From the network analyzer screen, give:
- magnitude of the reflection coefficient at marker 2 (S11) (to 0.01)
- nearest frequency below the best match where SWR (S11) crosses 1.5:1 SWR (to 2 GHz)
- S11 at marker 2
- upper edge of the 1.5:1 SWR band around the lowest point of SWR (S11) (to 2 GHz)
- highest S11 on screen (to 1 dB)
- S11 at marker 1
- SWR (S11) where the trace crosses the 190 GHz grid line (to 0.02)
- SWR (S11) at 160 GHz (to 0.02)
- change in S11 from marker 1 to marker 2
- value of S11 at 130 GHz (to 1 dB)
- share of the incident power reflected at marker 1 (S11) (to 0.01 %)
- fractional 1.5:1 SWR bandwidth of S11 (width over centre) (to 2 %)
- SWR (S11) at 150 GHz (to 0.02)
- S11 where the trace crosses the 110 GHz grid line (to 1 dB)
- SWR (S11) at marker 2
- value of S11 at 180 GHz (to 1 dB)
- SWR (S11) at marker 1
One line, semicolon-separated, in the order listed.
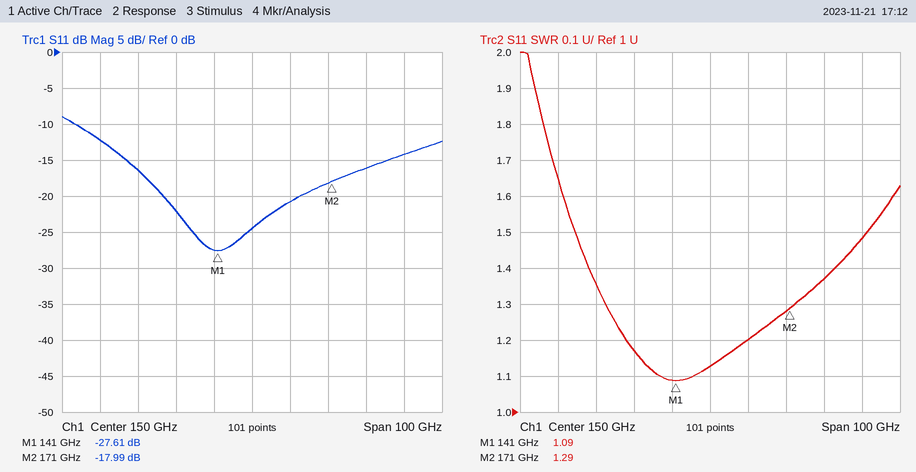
0.13; 114 GHz; -17.99 dB; 192 GHz; -9 dB; -27.61 dB; 1.48; 1.20; 9.62 dB; -22 dB; 0.17 %; 50 %; 1.12; -12 dB; 1.29; -16 dB; 1.09
